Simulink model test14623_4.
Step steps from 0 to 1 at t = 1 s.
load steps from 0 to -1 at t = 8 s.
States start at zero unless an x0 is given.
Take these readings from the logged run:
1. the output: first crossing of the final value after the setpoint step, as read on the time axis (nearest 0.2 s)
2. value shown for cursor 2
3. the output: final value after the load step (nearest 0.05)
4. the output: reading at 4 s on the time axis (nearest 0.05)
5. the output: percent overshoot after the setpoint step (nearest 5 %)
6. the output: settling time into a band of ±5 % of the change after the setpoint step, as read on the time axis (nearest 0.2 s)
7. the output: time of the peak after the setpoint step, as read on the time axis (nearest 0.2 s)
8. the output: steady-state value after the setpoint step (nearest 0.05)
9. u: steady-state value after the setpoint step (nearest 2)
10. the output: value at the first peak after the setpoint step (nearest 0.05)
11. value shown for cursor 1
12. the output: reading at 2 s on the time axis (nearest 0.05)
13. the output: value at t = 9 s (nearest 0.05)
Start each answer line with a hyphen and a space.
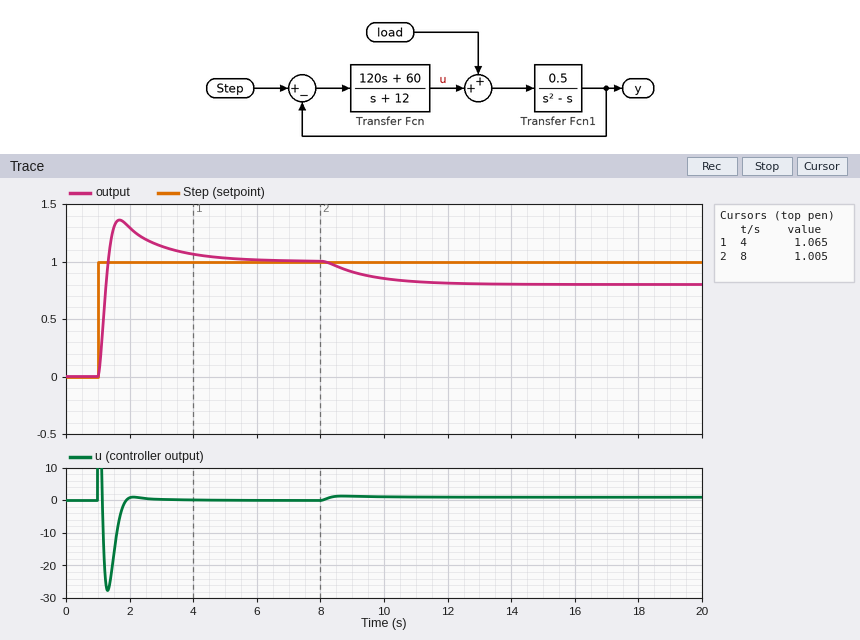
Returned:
- 1.4 s
- 1.005
- 0.80
- 1.05
- 35 %
- 4.4 s
- 1.6 s
- 1.00
- 0
- 1.35
- 1.065
- 1.30
- 0.90
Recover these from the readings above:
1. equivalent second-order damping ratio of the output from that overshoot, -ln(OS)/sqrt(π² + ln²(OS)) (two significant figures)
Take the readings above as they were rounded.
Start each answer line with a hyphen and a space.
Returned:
- 0.32
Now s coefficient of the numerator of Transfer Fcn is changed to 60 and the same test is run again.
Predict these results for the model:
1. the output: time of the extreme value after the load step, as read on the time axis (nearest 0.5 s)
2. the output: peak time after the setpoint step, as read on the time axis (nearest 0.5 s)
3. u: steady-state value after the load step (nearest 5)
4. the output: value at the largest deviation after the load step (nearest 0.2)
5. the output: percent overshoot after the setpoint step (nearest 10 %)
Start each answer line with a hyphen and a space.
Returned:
- 10.0 s
- 2.0 s
- 0
- 0.8
- 70 %
